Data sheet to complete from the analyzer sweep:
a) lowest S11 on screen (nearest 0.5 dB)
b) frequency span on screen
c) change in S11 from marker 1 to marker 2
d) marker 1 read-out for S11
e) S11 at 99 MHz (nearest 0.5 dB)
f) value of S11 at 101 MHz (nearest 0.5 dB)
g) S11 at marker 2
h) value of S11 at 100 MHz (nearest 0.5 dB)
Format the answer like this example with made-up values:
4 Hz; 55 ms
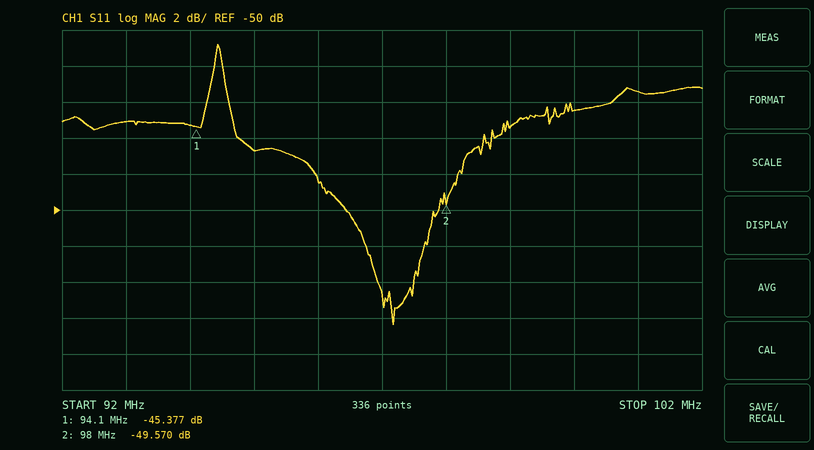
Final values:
-56.5 dB; 10 MHz; -4.193 dB; -45.377 dB; -45.5 dB; -43.5 dB; -49.570 dB; -44.5 dB
